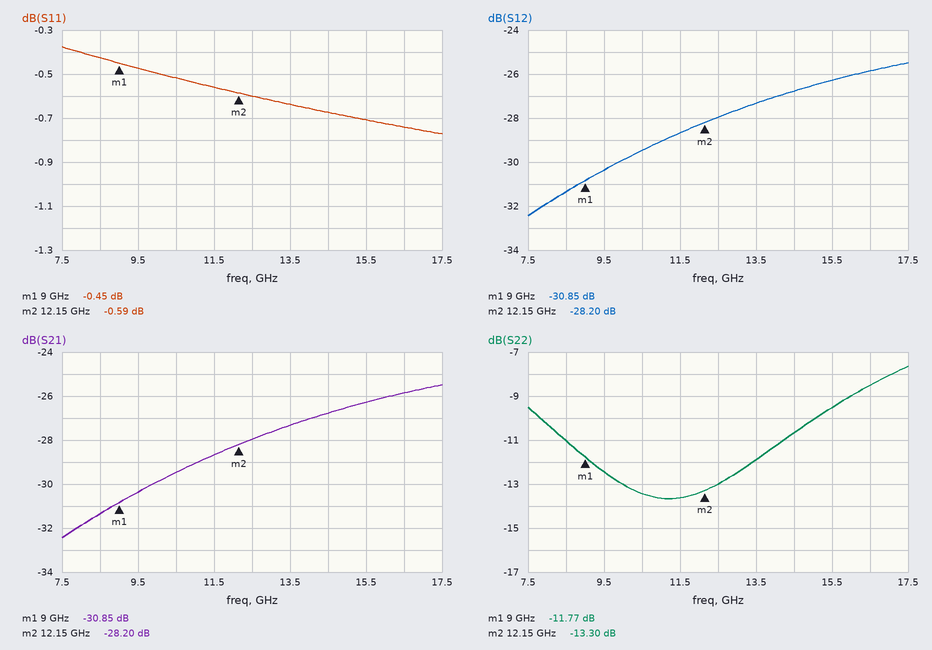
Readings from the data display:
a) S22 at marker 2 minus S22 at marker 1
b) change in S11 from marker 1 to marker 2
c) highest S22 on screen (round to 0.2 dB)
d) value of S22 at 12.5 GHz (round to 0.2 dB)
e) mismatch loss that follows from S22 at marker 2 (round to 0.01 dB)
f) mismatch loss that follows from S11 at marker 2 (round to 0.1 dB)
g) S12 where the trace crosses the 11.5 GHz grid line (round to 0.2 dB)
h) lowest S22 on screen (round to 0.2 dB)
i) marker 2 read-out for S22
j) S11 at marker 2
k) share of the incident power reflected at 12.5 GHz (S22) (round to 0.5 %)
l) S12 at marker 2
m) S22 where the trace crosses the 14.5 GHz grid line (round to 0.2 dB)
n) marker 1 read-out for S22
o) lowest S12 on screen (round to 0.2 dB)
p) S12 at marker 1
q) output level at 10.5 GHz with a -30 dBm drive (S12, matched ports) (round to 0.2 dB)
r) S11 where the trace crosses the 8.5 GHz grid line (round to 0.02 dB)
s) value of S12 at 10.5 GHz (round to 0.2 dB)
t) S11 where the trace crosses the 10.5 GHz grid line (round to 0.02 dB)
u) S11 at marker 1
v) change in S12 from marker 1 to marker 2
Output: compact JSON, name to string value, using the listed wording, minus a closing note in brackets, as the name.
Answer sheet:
{"S22 at marker 2 minus S22 at marker 1": "-1.53 dB", "change in S11 from marker 1 to marker 2": "-0.14 dB", "highest S22 on screen": "-7.6 dB", "value of S22 at 12.5 GHz": "-13.0 dB", "mismatch loss that follows from S22 at marker 2": "0.21 dB", "mismatch loss that follows from S11 at marker 2": "9.0 dB", "S12 where the trace crosses the 11.5 GHz grid line": "-28.6 dB", "lowest S22 on screen": "-13.6 dB", "marker 2 read-out for S22": "-13.30 dB", "S11 at marker 2": "-0.59 dB", "share of the incident power reflected at 12.5 GHz (S22)": "5.0 %", "S12 at marker 2": "-28.20 dB", "S22 where the trace crosses the 14.5 GHz grid line": "-10.6 dB", "marker 1 read-out for S22": "-11.77 dB", "lowest S12 on screen": "-32.4 dB", "S12 at marker 1": "-30.85 dB", "output level at 10.5 GHz with a -30 dBm drive (S12, matched ports)": "-59.4 dBm", "S11 where the trace crosses the 8.5 GHz grid line": "-0.42 dB", "value of S12 at 10.5 GHz": "-29.4 dB", "S11 where the trace crosses the 10.5 GHz grid line": "-0.52 dB", "S11 at marker 1": "-0.45 dB", "change in S12 from marker 1 to marker 2": "2.65 dB"}
